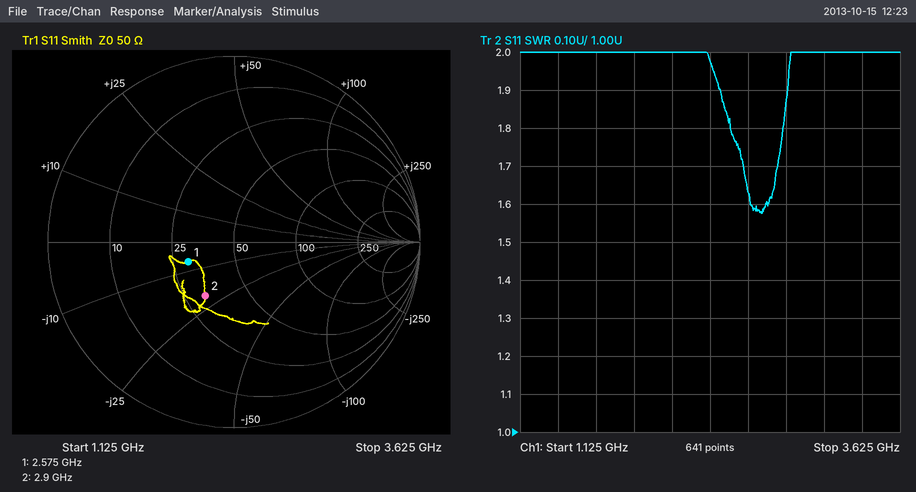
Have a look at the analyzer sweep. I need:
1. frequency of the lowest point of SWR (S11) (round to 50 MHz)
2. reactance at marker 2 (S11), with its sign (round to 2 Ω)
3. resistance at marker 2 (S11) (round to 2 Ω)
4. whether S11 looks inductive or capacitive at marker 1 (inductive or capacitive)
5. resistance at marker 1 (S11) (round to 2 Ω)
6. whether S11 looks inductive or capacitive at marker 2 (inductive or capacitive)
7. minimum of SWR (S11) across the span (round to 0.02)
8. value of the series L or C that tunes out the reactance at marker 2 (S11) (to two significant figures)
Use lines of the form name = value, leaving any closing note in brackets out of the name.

frequency of the lowest point of SWR (S11) = 2.70 GHz
reactance at marker 2 (S11), with its sign = -20 Ω
resistance at marker 2 (S11) = 32 Ω
whether S11 looks inductive or capacitive at marker 1 = capacitive
resistance at marker 1 (S11) = 30 Ω
whether S11 looks inductive or capacitive at marker 2 = capacitive
minimum of SWR (S11) across the span = 1.58
value of the series L or C that tunes out the reactance at marker 2 (S11) = 1.1 nH
